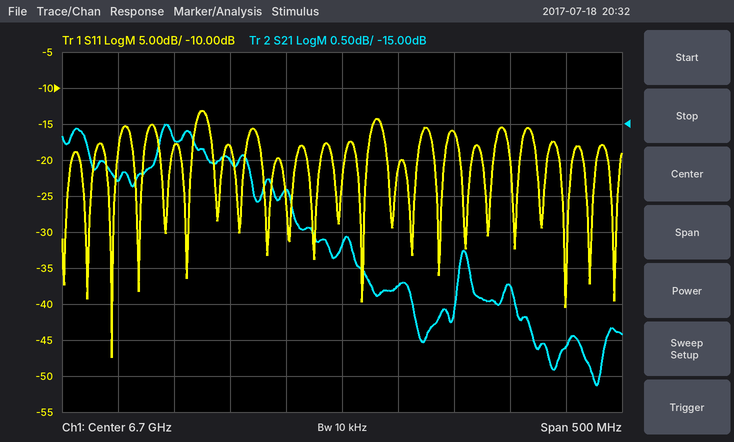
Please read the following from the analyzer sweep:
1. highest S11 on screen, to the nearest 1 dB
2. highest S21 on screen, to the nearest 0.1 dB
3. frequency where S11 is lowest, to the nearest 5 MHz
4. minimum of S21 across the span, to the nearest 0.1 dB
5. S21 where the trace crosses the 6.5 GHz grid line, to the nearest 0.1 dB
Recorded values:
-13 dB
-15.0 dB
6.495 GHz
-18.6 dB
-15.8 dB
